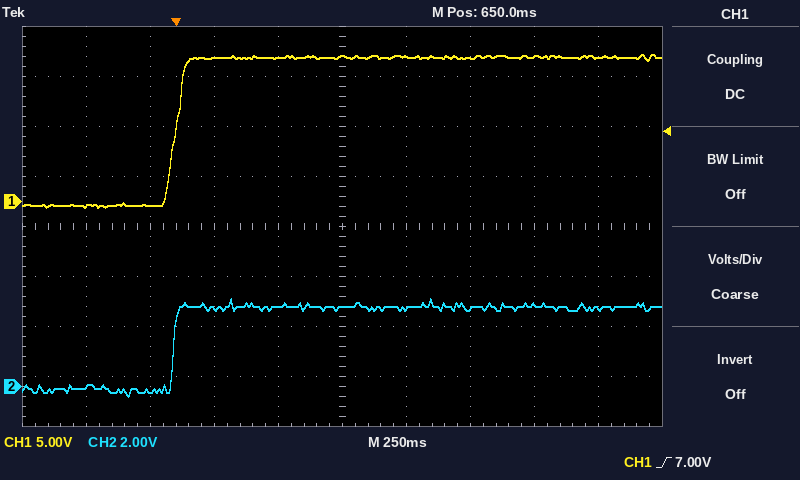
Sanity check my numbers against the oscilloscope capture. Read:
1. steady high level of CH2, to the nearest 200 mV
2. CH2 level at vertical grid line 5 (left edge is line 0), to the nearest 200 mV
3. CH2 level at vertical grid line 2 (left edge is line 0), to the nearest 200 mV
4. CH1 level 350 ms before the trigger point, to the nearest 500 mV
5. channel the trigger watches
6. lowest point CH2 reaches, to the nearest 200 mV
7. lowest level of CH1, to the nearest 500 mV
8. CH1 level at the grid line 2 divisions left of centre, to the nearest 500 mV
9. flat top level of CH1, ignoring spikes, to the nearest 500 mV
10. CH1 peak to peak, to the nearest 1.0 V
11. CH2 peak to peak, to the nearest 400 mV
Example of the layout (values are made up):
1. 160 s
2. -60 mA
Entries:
1. 3.2 V
2. 3.2 V
3. -200 mV
4. -500 mV
5. CH1
6. -400 mV
7. -500 mV
8. 14.5 V
9. 14.5 V
10. 15.0 V
11. 4.0 V
